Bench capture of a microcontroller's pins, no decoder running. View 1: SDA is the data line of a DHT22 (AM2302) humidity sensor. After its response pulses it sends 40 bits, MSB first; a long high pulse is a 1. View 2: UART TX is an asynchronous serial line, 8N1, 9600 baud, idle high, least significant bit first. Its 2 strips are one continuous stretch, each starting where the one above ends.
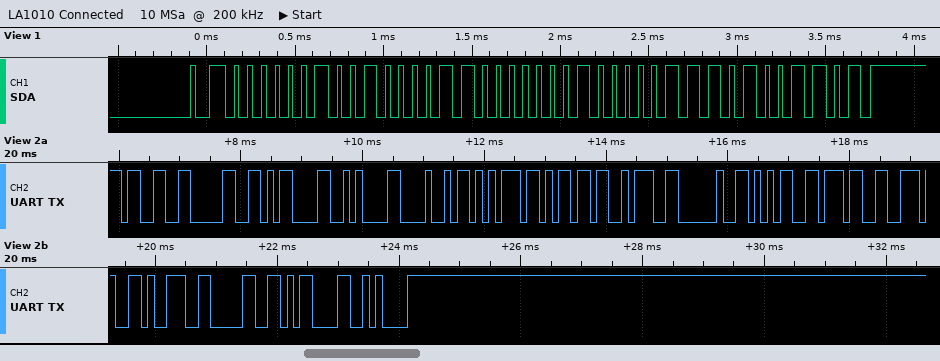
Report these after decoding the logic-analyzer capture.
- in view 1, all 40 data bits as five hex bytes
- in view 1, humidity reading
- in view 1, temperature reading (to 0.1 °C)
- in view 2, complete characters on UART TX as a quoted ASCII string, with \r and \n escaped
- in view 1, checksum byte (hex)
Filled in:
02 43 01 07 4D
57.9 %
26.3 °C
"30\r\nHum: 57.90\r\n"
0x4D
